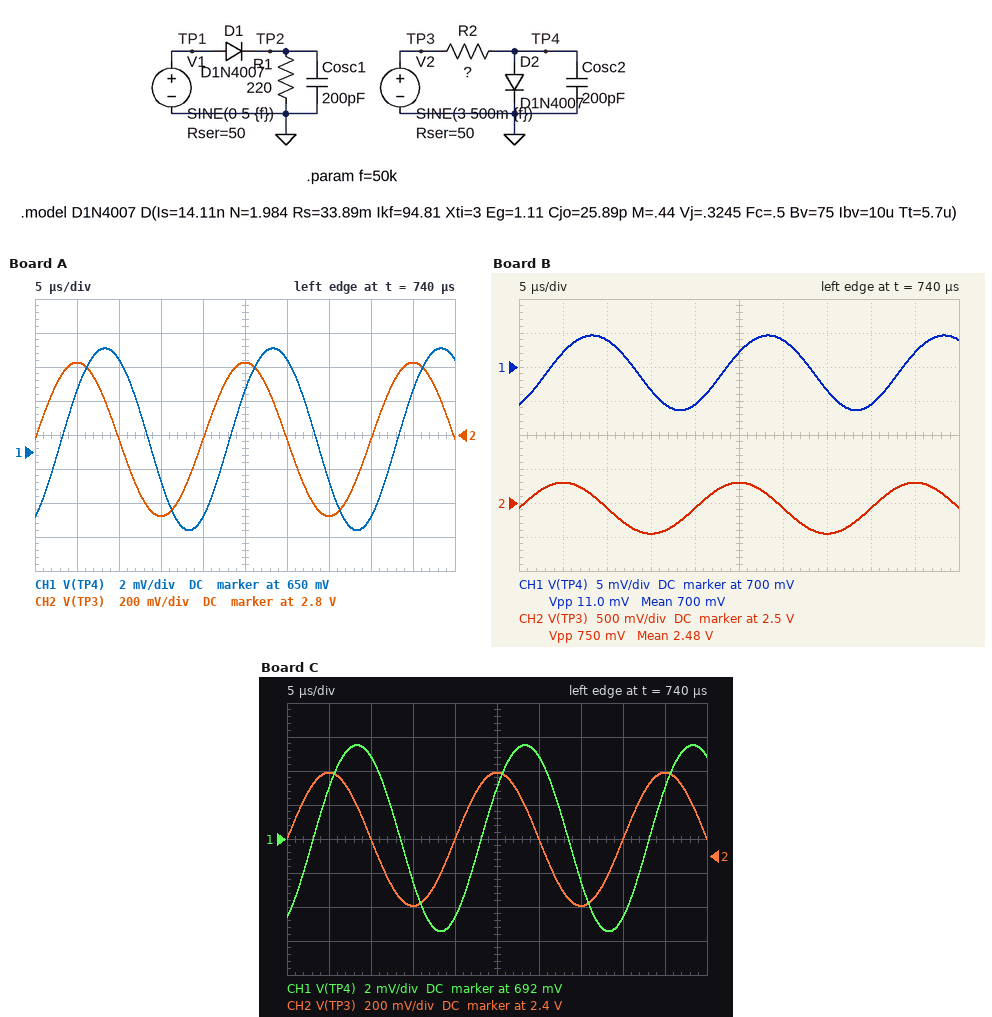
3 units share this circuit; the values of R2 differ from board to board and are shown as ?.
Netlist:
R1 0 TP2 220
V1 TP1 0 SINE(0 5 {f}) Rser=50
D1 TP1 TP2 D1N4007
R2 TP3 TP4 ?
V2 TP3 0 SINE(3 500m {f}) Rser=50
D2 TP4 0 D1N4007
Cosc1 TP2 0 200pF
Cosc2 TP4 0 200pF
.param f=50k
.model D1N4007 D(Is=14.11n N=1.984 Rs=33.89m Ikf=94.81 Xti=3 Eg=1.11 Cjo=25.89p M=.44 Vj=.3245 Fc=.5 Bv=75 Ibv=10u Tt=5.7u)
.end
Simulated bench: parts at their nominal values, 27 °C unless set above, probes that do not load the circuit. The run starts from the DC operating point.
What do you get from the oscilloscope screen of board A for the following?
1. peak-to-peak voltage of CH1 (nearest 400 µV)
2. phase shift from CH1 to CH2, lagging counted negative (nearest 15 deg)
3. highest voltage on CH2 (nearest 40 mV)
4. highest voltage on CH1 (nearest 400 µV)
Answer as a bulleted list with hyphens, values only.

- 10.8 mV
- 60 deg
- 3.24 V
- 656.0 mV
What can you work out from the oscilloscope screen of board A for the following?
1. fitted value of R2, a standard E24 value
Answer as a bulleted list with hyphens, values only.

- 470 Ω
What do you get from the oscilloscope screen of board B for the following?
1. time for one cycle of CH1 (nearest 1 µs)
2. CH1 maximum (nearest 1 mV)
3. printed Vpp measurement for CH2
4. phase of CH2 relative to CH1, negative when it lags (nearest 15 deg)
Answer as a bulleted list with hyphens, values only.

- 20 µs
- 705 mV
- 750 mV
- 60 deg
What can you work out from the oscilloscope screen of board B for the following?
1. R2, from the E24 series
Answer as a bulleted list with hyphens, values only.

- 150 Ω
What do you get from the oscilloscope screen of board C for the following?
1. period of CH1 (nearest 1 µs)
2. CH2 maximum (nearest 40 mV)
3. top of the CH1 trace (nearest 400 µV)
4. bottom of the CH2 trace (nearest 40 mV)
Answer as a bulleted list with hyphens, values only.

- 20 µs
- 2.88 V
- 697.6 mV
- 2.12 V
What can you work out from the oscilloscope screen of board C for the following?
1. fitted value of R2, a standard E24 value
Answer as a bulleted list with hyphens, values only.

- 180 Ω
